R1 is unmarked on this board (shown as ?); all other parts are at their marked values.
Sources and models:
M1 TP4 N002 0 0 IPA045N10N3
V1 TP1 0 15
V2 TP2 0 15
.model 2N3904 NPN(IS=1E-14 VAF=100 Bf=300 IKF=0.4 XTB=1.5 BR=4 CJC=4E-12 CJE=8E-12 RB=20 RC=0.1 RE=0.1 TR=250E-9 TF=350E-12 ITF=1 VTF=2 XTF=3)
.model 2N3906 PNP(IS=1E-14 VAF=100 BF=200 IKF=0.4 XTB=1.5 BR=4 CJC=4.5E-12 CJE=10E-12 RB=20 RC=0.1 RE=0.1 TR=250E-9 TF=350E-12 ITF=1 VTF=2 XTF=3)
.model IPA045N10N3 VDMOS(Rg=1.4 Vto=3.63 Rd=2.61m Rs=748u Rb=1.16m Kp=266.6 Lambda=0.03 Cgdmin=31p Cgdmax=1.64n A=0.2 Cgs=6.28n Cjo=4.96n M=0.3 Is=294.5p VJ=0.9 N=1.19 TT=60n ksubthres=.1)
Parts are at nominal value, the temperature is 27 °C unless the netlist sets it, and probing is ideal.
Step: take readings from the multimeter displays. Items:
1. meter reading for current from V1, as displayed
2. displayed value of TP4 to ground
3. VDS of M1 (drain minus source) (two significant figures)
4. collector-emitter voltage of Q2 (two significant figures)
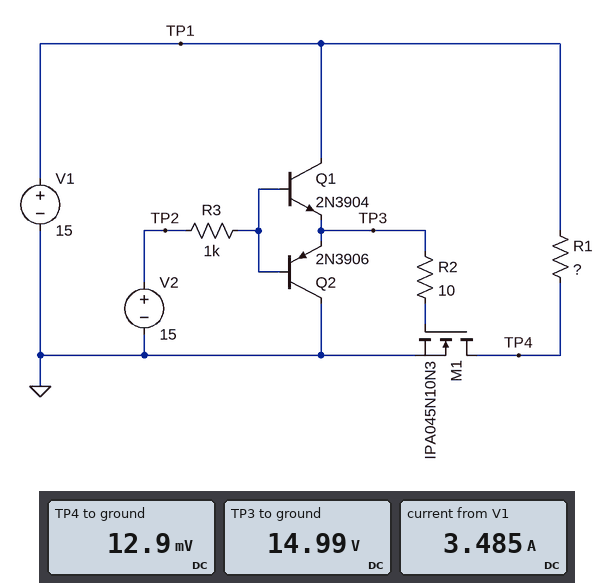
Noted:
3.485 A
12.9 mV
13 mV
-15 V
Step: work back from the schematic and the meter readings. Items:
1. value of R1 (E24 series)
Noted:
4.3 Ω
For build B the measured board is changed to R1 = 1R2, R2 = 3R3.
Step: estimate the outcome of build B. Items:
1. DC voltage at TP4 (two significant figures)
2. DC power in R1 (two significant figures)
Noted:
46 mV
190 W
